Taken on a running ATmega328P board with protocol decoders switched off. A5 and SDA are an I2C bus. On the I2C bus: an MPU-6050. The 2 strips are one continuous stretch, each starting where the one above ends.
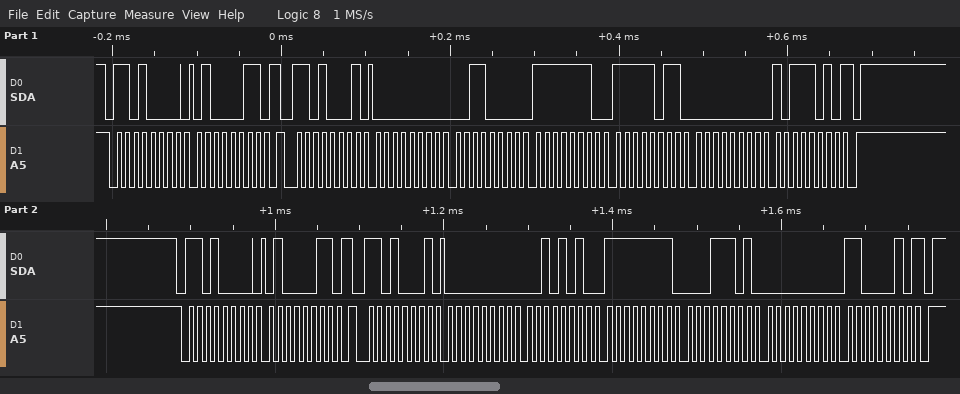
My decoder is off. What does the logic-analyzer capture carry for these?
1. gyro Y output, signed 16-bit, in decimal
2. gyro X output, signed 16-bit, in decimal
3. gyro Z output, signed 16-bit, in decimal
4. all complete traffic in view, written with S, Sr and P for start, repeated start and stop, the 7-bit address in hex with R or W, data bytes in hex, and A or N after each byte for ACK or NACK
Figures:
-261
48
186
S 68W A 43 A Sr 68R A 00 A 30 A FE A FB A 00 A BA N P S 68W A 43 A Sr 68R A 00 A 2A A FF A 1D A 00 A C2 N P
